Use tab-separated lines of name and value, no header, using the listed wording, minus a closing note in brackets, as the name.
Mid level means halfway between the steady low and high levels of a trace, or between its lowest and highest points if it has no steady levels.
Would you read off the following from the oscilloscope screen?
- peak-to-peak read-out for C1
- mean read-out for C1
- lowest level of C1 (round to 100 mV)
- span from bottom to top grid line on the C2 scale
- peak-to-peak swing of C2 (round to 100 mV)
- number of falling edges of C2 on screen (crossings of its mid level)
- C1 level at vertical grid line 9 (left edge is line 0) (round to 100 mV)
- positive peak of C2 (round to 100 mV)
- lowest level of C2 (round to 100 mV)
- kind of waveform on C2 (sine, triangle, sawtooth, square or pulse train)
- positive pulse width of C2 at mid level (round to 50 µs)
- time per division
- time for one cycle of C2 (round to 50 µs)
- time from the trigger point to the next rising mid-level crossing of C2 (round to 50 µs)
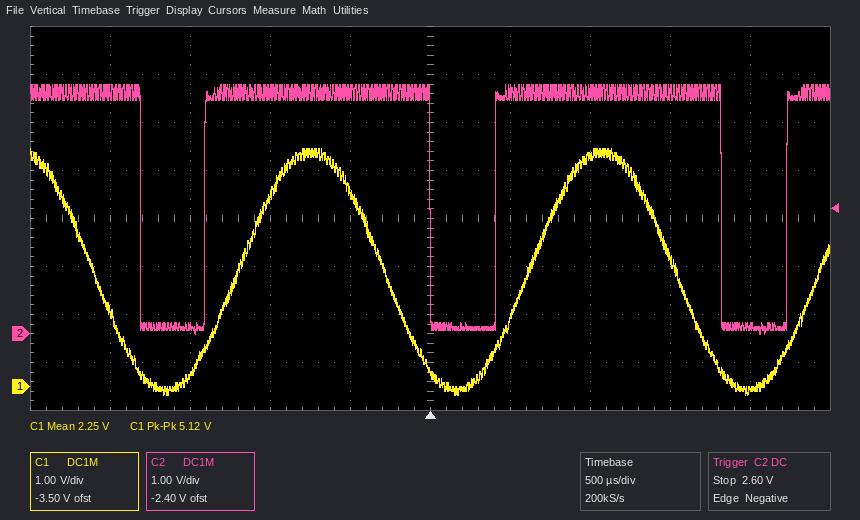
peak-to-peak read-out for C1	5.12 V
mean read-out for C1	2.25 V
lowest level of C1	-200 mV
span from bottom to top grid line on the C2 scale	8 V
peak-to-peak swing of C2	5.2 V
number of falling edges of C2 on screen	3
C1 level at vertical grid line 9 (left edge is line 0)	-100 mV
positive peak of C2	5.2 V
lowest level of C2	0.0 V
kind of waveform on C2	pulse train
positive pulse width of C2 at mid level	1.40 ms
time per division	500 µs
time for one cycle of C2	1.80 ms
time from the trigger point to the next rising mid-level crossing of C2	400 µs
